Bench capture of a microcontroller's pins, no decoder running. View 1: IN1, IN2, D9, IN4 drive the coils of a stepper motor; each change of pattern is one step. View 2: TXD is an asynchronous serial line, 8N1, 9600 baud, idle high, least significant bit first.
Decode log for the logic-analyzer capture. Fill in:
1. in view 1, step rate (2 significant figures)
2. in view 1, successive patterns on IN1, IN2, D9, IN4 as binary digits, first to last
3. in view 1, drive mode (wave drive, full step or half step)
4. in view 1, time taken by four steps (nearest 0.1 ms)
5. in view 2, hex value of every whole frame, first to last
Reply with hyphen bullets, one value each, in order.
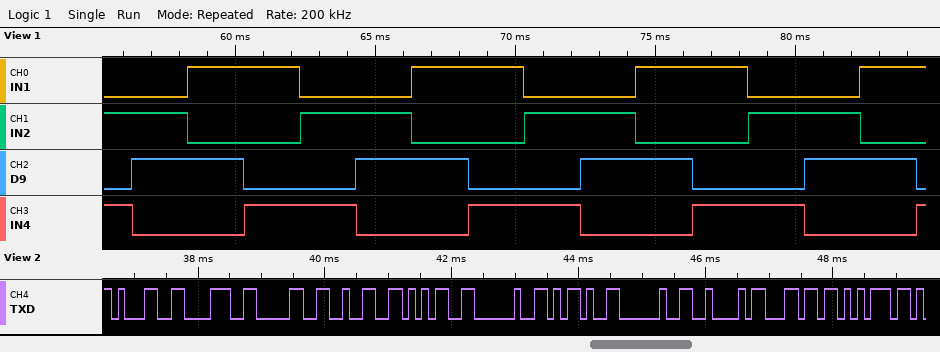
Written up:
- 500 steps/s
- 0101 0110 1010 1001 0101 0110 1010 1001 0101 0110 1010 1001 0101 0110 1010 1001
- full step
- 8.0 ms
- 31 38 30 32 35 20 2D 20 42 6C 75
